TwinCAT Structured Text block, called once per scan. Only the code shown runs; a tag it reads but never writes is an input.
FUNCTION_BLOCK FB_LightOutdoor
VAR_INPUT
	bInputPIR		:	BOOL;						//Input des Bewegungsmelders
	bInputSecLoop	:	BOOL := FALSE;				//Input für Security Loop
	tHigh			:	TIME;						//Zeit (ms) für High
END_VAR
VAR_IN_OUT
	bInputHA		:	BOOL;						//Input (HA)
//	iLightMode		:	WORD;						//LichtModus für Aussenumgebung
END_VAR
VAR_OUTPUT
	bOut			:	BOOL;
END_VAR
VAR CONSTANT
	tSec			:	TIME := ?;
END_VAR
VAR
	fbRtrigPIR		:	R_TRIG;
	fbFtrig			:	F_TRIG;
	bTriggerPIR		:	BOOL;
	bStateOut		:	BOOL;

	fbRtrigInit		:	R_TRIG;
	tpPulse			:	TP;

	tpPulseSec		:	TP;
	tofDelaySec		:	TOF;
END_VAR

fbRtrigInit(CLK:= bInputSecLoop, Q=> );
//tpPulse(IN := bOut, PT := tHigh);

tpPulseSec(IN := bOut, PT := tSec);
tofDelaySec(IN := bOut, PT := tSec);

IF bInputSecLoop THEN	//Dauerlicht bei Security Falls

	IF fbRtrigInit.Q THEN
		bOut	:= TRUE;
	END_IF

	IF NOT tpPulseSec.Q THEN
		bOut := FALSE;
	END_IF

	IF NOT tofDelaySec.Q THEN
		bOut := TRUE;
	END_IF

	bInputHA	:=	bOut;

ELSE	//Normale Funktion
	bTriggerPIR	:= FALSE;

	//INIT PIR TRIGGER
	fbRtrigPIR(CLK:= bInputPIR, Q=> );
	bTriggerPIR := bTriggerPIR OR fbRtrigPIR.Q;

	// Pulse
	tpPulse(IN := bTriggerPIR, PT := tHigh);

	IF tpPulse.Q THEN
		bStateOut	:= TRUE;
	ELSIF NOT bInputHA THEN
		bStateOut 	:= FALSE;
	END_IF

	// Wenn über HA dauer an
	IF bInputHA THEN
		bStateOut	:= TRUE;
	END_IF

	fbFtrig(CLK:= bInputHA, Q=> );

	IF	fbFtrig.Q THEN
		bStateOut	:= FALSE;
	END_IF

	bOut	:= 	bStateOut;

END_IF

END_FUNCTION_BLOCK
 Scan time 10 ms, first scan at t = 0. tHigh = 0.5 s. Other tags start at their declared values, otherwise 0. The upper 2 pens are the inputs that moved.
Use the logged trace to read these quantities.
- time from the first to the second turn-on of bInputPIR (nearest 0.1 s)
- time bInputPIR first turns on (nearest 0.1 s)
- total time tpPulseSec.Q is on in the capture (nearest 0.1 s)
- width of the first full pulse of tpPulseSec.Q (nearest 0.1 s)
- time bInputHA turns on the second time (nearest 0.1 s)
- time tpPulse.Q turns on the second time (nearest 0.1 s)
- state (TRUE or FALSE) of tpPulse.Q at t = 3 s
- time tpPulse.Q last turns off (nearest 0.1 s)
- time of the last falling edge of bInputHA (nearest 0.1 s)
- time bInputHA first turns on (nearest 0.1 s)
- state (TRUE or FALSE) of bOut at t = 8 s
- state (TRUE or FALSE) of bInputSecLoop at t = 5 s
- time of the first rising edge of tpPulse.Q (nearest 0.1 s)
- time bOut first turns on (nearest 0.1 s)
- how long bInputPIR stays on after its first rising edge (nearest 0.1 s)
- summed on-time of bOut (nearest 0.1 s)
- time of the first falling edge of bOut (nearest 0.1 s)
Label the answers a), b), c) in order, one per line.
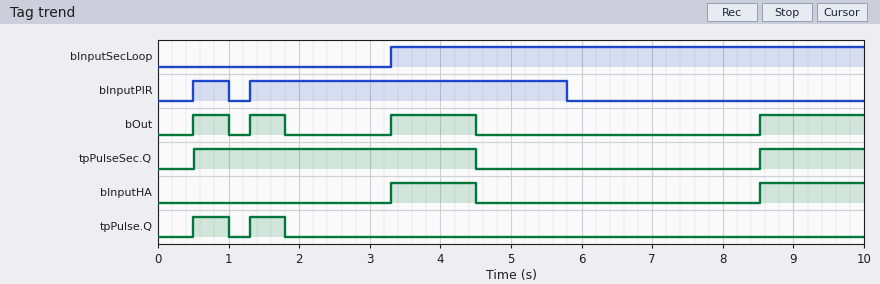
a) 0.8 s
b) 0.5 s
c) 5.5 s
d) 4.0 s
e) 8.5 s
f) 1.3 s
g) FALSE
h) 1.8 s
i) 4.5 s
j) 3.3 s
k) FALSE
l) TRUE
m) 0.5 s
n) 0.5 s
o) 0.5 s
p) 3.7 s
q) 1.0 s
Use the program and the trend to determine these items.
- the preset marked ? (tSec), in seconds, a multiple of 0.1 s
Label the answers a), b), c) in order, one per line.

a) 4.0 s
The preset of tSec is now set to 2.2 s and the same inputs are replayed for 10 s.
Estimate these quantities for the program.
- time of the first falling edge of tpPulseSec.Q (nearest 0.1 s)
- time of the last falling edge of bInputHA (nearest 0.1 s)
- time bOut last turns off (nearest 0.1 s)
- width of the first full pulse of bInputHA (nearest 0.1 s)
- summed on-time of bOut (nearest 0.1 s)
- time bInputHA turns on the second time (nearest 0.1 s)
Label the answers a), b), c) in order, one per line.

a) 2.7 s
b) 6.2 s
c) 6.2 s
d) 2.2 s
e) 4.8 s
f) 8.4 s
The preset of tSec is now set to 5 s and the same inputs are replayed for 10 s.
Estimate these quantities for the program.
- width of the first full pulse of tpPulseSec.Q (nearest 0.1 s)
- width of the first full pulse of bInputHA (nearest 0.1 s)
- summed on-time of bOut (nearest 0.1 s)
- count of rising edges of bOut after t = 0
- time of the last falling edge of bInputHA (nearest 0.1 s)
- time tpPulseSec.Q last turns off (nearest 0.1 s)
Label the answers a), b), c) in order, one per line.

a) 5.0 s
b) 2.2 s
c) 3.2 s
d) 3
e) 5.5 s
f) 5.5 s
